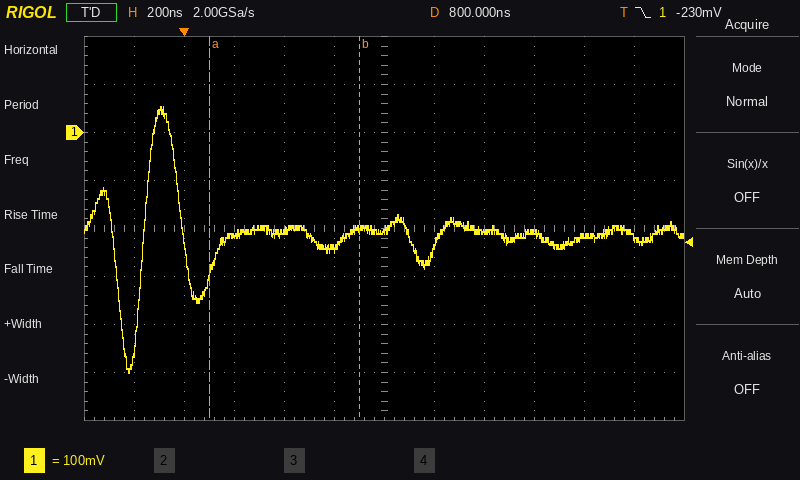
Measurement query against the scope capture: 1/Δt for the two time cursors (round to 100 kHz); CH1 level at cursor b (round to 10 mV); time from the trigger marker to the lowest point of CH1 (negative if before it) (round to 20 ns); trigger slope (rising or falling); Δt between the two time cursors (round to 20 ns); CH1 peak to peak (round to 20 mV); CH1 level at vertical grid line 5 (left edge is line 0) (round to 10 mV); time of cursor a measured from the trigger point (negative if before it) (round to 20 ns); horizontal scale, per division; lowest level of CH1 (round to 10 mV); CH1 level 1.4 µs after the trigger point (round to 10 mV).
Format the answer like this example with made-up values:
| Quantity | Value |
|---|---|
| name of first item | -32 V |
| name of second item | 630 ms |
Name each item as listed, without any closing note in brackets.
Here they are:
| Quantity | Value |
|---|---|
| 1/Δt for the two time cursors | 1.7 MHz |
| CH1 level at cursor b | -200 mV |
| time from the trigger marker to the lowest point of CH1 (negative if before it) | -220 ns |
| trigger slope | falling |
| Δt between the two time cursors | 600 ns |
| CH1 peak to peak | 560 mV |
| CH1 level at vertical grid line 5 (left edge is line 0) | -240 mV |
| time of cursor a measured from the trigger point (negative if before it) | +100 ns |
| horizontal scale, per division | 200 ns |
| lowest level of CH1 | -500 mV |
| CH1 level 1.4 µs after the trigger point | -210 mV |
